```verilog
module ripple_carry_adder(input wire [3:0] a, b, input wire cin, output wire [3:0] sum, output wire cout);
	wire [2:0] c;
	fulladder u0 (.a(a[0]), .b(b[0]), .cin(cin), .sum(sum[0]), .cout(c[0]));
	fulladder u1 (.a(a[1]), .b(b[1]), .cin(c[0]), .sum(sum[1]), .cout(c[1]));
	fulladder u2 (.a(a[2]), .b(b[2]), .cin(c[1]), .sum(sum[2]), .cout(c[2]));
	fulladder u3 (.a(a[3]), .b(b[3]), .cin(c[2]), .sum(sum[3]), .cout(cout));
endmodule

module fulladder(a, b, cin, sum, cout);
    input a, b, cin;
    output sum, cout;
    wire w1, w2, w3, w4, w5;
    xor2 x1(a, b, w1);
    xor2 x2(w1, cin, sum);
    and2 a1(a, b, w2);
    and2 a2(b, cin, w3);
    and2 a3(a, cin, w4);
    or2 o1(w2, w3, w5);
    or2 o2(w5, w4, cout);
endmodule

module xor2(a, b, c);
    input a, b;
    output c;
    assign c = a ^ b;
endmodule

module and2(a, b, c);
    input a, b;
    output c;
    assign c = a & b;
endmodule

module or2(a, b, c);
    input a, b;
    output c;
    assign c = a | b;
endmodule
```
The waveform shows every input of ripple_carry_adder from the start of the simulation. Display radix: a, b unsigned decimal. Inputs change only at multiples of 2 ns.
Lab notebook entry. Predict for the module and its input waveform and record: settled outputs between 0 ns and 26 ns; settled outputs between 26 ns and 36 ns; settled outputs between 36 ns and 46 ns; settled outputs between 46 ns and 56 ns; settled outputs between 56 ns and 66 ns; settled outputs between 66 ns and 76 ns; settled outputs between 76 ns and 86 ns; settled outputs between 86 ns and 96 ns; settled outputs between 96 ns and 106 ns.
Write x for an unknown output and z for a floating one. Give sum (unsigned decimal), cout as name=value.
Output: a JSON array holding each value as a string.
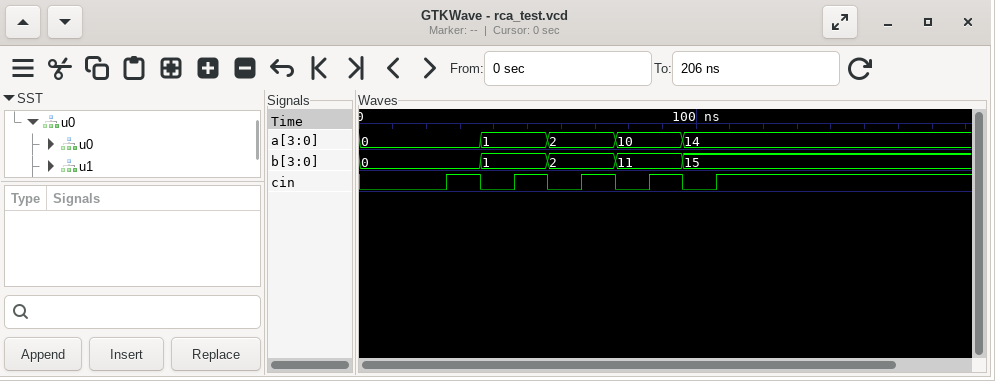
["sum=0, cout=0", "sum=1, cout=0", "sum=2, cout=0", "sum=3, cout=0", "sum=4, cout=0", "sum=5, cout=0", "sum=5, cout=1", "sum=6, cout=1", "sum=13, cout=1"]
